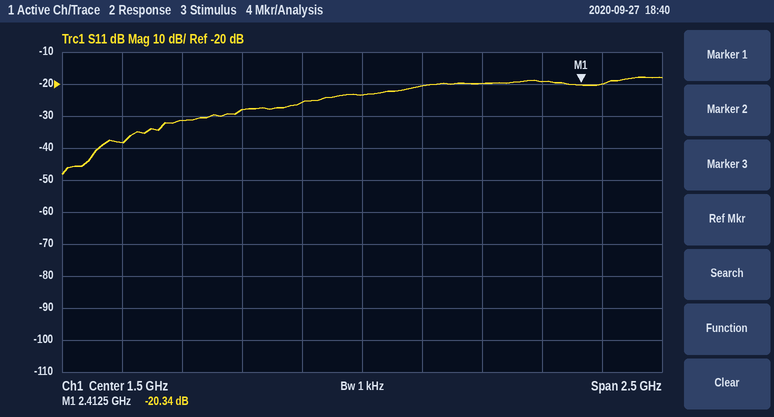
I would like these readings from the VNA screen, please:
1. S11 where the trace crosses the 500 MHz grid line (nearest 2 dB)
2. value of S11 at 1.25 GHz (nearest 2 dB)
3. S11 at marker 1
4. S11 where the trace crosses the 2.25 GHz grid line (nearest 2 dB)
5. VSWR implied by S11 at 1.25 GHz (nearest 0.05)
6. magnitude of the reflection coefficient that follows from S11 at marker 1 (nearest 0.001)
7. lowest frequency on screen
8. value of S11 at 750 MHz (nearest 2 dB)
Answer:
-38 dB
-26 dB
-20.34 dB
-20 dB
1.10
0.096
250 MHz
-32 dB
